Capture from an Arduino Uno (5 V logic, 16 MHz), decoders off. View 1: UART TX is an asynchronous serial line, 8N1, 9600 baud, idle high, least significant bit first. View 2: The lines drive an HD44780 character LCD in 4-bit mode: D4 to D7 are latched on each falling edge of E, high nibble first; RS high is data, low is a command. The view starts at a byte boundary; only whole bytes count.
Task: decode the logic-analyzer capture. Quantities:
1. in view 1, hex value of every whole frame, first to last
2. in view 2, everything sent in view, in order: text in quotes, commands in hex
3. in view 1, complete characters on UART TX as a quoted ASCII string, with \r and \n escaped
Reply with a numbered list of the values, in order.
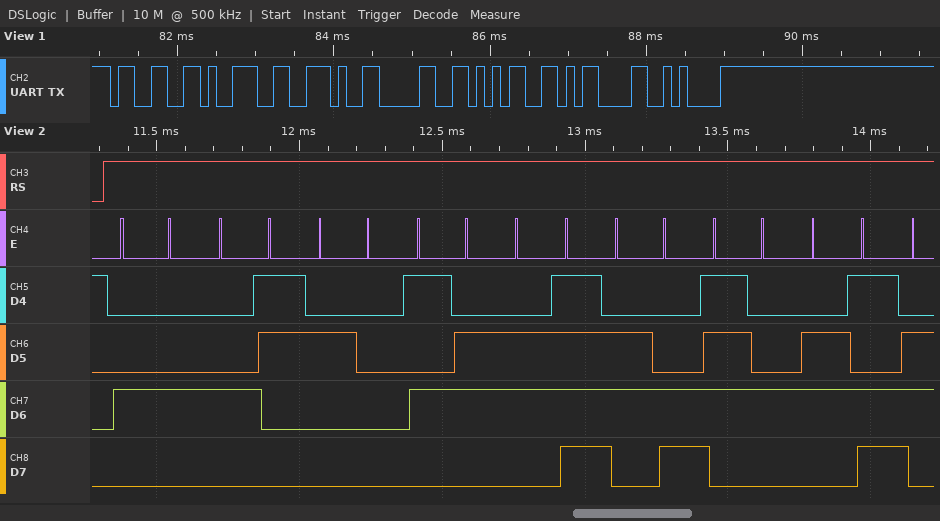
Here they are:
1. 0x33 0x39 0x2E 0x30 0x35 0x0D 0x0A
2. "DC Voltm"
3. "39.05\r\n"
